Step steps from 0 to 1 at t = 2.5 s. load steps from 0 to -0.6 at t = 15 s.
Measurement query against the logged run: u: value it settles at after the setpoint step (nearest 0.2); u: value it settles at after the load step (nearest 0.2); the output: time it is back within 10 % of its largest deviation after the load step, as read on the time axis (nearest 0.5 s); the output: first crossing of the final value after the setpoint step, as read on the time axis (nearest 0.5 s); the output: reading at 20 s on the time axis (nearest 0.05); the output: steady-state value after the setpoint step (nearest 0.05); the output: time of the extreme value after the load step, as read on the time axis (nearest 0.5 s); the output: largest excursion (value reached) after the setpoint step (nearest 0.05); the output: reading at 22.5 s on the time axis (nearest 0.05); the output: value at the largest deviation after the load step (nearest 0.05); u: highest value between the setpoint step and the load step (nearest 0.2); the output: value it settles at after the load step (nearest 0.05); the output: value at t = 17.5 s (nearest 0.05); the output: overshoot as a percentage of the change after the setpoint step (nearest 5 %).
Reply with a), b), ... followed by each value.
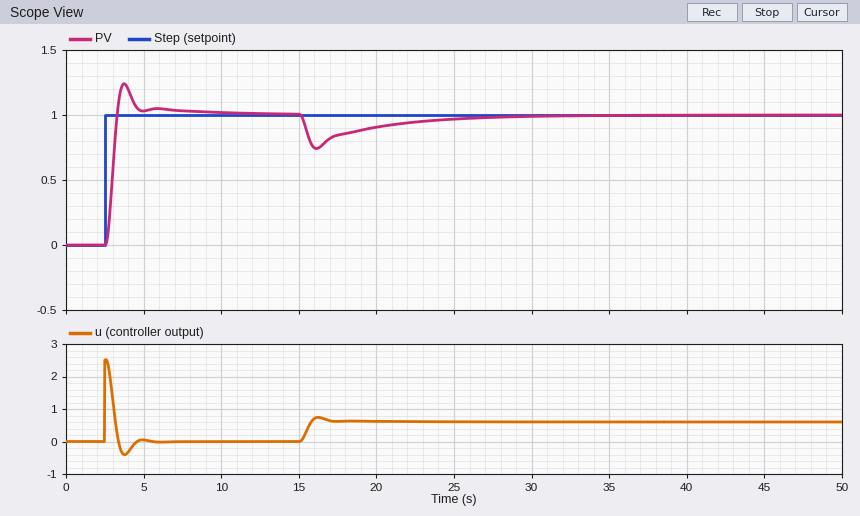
a) 0.0
b) 0.6
c) 26.0 s
d) 3.5 s
e) 0.90
f) 1.00
g) 16.0 s
h) 1.25
i) 0.95
j) 0.75
k) 2.6
l) 1.00
m) 0.85
n) 25 %
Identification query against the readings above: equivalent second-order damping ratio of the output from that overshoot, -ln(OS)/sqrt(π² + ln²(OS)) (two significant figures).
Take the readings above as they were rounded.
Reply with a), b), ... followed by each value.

a) 0.40
